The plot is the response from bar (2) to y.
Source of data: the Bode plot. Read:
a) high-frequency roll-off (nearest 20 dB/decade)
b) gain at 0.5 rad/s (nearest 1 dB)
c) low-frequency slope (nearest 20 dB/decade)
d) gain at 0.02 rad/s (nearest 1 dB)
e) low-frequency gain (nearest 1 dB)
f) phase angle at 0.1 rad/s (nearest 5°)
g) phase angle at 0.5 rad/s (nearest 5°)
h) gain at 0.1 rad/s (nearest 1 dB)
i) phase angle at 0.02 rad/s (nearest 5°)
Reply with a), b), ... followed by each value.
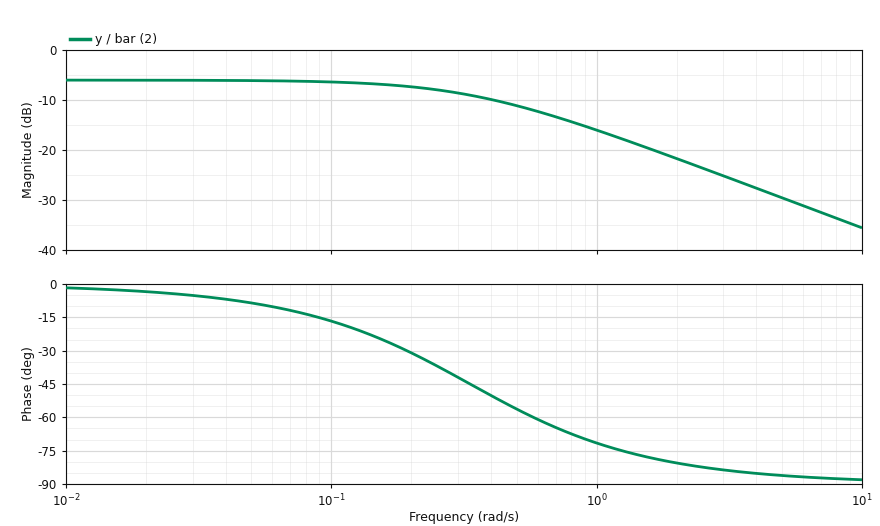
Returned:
a) -20 dB/decade
b) -11 dB
c) 0 dB/decade
d) -6 dB
e) -6 dB
f) -15°
g) -55°
h) -6 dB
i) -5°
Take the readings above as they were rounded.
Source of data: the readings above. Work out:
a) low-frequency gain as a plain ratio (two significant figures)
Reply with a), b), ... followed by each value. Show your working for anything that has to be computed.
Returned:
a) 10^(-6 / 20) = 0.50
